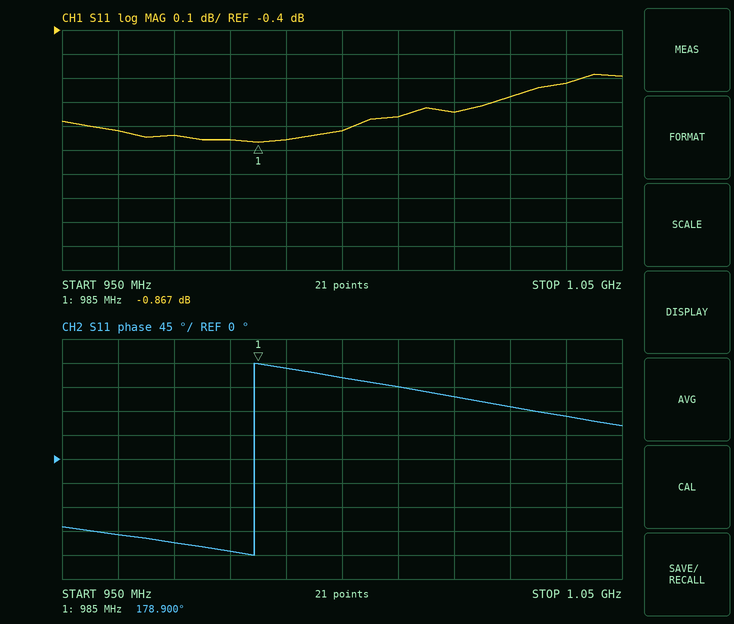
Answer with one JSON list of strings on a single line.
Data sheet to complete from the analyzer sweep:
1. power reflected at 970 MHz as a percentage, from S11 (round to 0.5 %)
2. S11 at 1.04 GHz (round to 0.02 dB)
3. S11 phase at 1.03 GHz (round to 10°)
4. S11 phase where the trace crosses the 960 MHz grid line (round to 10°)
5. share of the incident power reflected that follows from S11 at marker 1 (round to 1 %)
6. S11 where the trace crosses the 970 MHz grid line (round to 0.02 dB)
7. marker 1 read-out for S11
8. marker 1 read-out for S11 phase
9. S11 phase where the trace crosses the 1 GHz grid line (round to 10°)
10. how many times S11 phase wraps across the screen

["82.5 %", "-0.62 dB", "100°", "-140°", "82 %", "-0.84 dB", "-0.867 dB", "178.900°", "150°", "1"]
